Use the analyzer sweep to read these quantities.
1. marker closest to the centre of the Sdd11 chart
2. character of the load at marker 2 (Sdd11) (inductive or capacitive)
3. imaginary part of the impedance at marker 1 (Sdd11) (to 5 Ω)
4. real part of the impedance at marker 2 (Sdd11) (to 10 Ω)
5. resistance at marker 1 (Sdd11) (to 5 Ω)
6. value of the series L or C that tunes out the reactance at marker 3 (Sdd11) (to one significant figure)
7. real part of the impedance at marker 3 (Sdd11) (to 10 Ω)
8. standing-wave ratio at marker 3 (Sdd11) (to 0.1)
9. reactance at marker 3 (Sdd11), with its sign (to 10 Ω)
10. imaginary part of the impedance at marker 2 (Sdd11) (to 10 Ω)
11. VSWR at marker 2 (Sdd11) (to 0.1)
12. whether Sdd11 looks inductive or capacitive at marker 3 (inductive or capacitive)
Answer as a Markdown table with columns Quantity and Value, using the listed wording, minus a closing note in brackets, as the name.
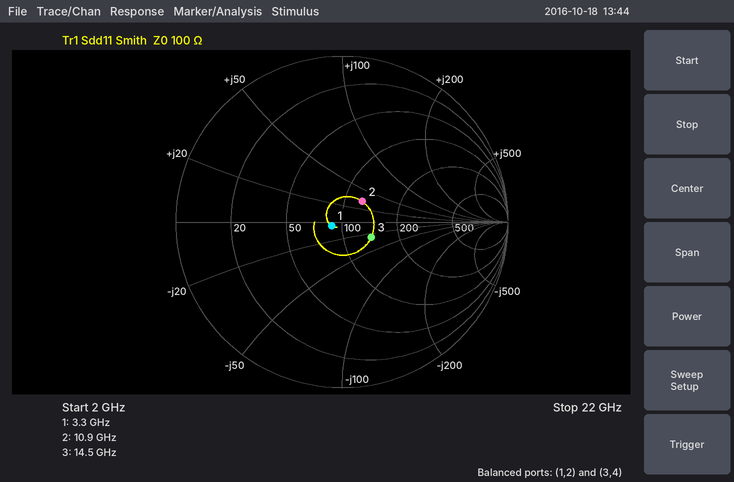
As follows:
| Quantity | Value |
|---|---|
| marker closest to the centre of the Sdd11 chart | marker 1 |
| character of the load at marker 2 (Sdd11) | inductive |
| imaginary part of the impedance at marker 1 (Sdd11) | -5 Ω |
| real part of the impedance at marker 2 (Sdd11) | 120 Ω |
| resistance at marker 1 (Sdd11) | 90 Ω |
| value of the series L or C that tunes out the reactance at marker 3 (Sdd11) | 300 pH |
| real part of the impedance at marker 3 (Sdd11) | 140 Ω |
| standing-wave ratio at marker 3 (Sdd11) | 1.5 |
| reactance at marker 3 (Sdd11), with its sign | -30 Ω |
| imaginary part of the impedance at marker 2 (Sdd11) | +30 Ω |
| VSWR at marker 2 (Sdd11) | 1.4 |
| whether Sdd11 looks inductive or capacitive at marker 3 | capacitive |
